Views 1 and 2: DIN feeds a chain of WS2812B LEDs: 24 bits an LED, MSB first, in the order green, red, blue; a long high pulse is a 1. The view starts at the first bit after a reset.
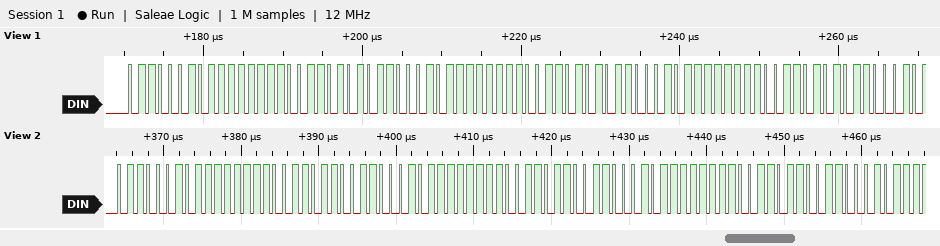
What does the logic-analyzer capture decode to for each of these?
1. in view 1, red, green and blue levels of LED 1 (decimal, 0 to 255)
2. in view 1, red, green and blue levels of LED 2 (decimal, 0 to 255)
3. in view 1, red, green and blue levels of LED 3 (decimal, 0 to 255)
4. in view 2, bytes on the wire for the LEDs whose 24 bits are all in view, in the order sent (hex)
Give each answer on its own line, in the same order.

255, 98, 53
255, 98, 53
255, 98, 53
62 FF 36 62 FF 36 62 FF 36
